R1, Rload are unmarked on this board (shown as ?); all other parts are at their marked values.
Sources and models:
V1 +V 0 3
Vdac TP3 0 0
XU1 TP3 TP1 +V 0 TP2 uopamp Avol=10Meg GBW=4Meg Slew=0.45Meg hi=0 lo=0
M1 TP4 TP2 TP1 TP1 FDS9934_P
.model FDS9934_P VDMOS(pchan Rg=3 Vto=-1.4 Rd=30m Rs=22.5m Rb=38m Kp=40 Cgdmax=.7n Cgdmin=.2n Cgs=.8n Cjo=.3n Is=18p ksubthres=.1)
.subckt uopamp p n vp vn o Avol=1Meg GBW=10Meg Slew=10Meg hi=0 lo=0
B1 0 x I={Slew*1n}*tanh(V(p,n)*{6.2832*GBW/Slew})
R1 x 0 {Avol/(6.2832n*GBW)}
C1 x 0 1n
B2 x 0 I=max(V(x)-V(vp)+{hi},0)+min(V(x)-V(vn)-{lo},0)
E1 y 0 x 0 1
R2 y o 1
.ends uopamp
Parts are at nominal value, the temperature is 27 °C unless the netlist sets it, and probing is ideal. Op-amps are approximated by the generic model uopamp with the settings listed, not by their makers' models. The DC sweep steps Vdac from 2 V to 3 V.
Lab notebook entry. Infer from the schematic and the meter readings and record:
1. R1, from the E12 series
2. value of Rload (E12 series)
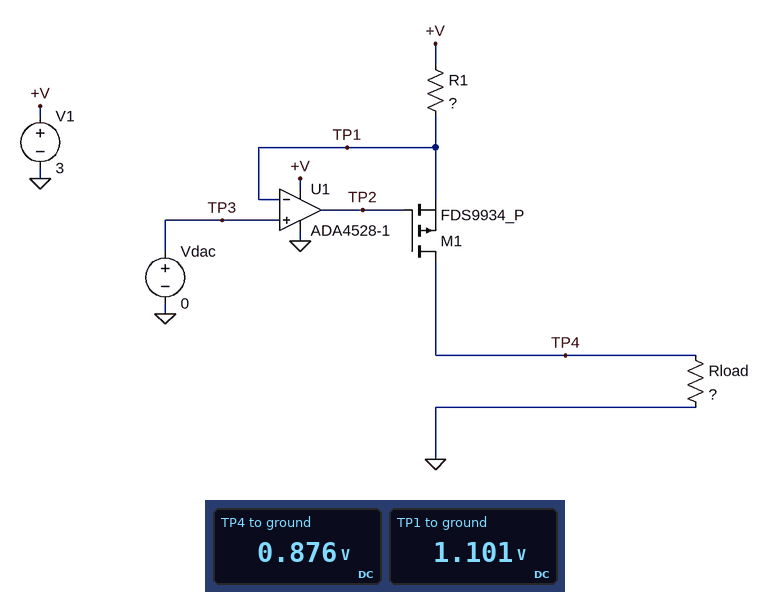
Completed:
3.9 kΩ
1.8 kΩ
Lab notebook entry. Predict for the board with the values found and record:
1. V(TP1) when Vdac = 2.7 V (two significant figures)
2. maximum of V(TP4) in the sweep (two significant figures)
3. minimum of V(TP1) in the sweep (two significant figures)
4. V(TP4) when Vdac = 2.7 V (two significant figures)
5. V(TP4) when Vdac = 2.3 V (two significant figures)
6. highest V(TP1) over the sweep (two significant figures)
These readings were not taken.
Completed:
2.7 V
460 mV
2.0 V
140 mV
320 mV
3.0 V
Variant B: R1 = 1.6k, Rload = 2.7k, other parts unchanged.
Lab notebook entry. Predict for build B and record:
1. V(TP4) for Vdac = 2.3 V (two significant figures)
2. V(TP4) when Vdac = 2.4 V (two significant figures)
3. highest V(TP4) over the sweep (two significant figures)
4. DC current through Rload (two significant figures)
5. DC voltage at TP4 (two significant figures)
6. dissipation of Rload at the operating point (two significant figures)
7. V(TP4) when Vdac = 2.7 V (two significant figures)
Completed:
1.2 V
1.0 V
1.7 V
700 µA
1.9 V
1.3 mW
510 mV
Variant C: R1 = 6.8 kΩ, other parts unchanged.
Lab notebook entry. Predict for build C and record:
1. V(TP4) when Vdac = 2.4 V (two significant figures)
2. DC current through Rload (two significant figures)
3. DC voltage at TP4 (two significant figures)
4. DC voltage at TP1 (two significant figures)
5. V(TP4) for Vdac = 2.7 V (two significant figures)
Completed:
160 mV
280 µA
510 mV
1.1 V
79 mV
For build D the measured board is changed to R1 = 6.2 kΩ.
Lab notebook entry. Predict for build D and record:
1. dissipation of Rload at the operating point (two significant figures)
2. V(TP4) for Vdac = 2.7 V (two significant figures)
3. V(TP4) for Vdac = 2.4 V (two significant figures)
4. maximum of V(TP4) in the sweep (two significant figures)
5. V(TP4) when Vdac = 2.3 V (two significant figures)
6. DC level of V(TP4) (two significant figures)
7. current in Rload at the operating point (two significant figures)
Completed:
170 µW
87 mV
170 mV
290 mV
200 mV
560 mV
310 µA
